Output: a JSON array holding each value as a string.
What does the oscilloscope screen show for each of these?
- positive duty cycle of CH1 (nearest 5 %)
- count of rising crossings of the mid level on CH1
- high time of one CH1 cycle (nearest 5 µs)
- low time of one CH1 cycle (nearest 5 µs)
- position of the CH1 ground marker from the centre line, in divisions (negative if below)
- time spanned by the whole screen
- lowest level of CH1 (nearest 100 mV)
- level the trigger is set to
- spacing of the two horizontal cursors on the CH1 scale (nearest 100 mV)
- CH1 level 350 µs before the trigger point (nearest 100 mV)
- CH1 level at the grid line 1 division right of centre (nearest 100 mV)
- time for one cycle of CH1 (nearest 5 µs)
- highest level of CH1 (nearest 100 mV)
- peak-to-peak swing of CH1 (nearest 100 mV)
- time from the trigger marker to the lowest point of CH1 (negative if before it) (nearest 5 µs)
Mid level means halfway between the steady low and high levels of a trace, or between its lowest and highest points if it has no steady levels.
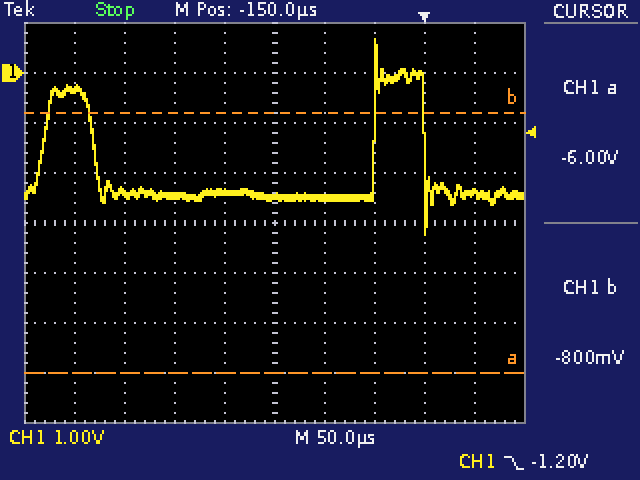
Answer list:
["15 %", "2", "50 µs", "280 µs", "+3.0 div", "500 µs", "-3.2 V", "-1.20 V", "5.2 V", "-300 mV", "-2.5 V", "330 µs", "700 mV", "3.9 V", "0 µs"]
